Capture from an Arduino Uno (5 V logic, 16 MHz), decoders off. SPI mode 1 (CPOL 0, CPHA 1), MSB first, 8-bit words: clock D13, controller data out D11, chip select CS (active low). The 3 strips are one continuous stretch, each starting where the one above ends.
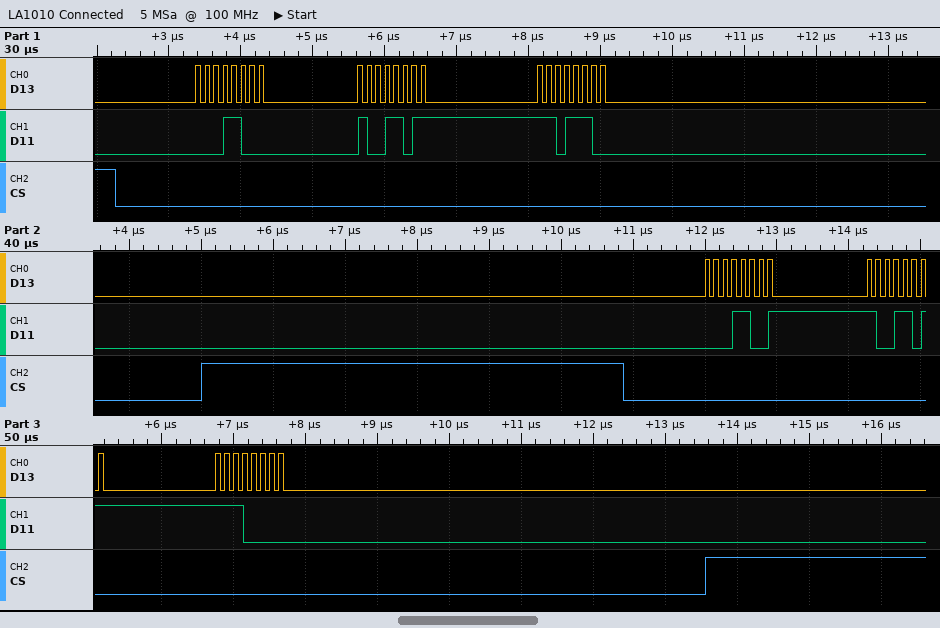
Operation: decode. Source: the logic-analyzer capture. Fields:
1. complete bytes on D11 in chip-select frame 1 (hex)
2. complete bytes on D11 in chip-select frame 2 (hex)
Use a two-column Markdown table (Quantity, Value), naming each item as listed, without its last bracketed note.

| Quantity | Value |
|---|---|
| complete bytes on D11 in chip-select frame 1 | 0x18 0x9B 0xDC |
| complete bytes on D11 in chip-select frame 2 | 0x19 0x9B 0xE0 |
